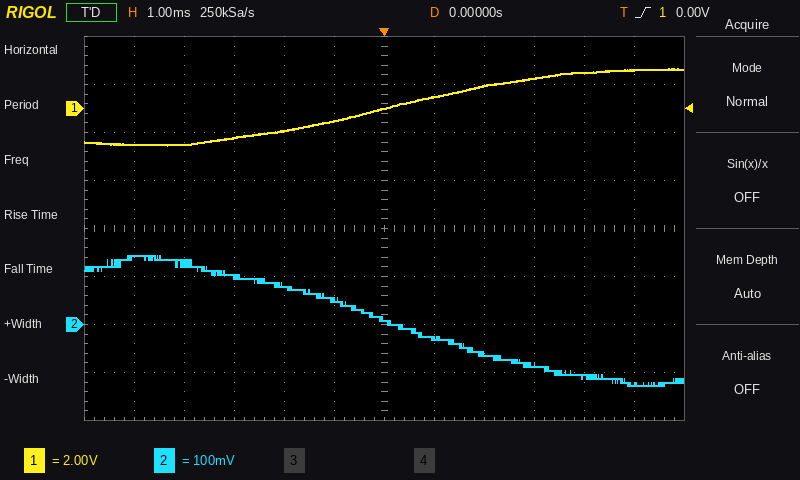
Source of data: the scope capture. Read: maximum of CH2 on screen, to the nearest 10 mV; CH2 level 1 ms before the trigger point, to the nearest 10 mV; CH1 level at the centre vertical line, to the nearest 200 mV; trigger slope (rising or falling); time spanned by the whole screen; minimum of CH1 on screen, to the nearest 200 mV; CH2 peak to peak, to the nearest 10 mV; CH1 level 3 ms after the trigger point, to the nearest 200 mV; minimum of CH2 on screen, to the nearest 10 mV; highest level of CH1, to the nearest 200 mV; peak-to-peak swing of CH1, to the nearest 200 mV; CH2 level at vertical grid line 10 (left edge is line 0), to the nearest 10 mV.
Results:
140 mV
50 mV
0.0 V
rising
12 ms
-1.6 V
270 mV
1.2 V
-130 mV
1.6 V
3.2 V
-110 mV
